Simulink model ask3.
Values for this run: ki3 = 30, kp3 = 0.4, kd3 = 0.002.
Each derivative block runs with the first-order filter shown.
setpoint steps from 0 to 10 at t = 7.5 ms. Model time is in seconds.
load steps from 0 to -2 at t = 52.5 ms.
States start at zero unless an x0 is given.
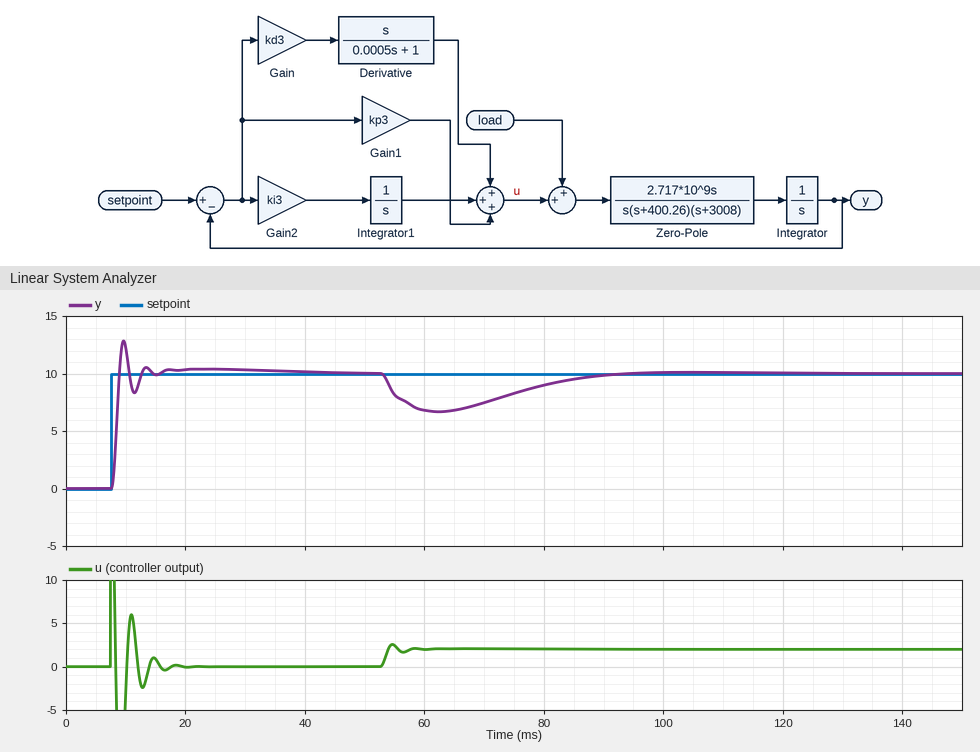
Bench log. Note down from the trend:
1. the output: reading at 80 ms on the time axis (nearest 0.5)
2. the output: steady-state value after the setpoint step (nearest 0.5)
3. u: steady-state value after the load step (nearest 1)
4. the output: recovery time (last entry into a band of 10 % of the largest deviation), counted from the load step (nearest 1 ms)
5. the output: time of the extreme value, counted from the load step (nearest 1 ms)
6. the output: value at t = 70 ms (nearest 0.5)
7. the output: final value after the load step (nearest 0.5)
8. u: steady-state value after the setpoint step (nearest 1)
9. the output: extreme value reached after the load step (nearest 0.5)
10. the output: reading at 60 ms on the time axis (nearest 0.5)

9.0
10.0
2
35 ms
10 ms
7.5
10.0
0
6.5
7.0
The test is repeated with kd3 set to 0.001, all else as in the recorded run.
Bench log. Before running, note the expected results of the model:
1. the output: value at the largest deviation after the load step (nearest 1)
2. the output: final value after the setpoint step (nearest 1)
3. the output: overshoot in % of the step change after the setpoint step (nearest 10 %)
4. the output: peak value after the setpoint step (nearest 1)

6
10
20 %
12
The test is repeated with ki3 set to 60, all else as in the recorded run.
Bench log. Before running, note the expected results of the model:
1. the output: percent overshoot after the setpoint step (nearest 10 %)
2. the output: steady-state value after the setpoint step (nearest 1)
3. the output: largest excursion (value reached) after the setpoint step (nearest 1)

30 %
10
13
